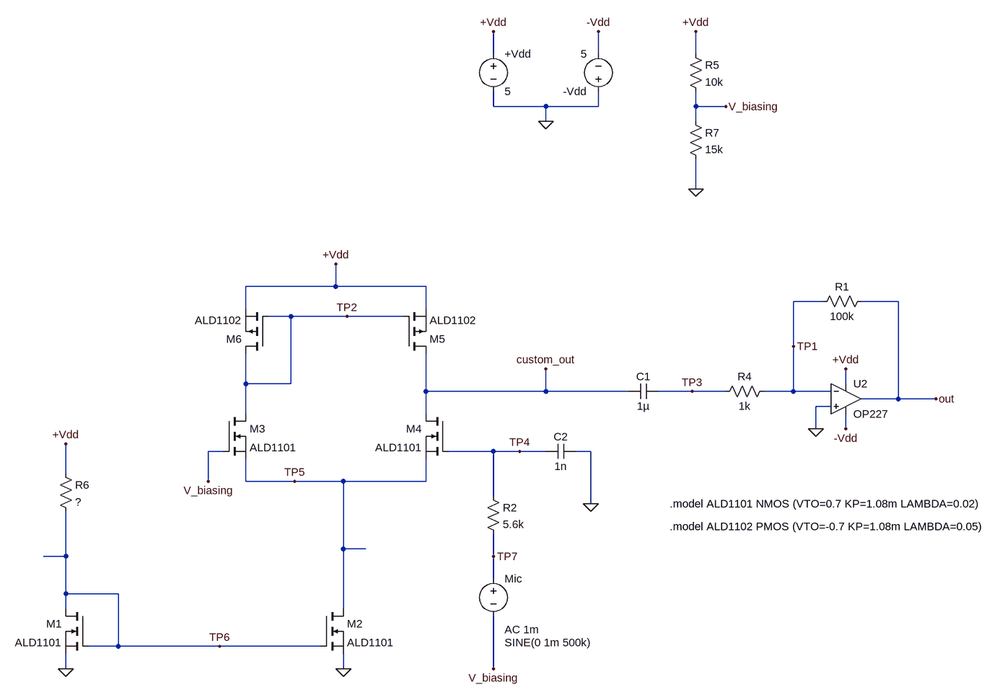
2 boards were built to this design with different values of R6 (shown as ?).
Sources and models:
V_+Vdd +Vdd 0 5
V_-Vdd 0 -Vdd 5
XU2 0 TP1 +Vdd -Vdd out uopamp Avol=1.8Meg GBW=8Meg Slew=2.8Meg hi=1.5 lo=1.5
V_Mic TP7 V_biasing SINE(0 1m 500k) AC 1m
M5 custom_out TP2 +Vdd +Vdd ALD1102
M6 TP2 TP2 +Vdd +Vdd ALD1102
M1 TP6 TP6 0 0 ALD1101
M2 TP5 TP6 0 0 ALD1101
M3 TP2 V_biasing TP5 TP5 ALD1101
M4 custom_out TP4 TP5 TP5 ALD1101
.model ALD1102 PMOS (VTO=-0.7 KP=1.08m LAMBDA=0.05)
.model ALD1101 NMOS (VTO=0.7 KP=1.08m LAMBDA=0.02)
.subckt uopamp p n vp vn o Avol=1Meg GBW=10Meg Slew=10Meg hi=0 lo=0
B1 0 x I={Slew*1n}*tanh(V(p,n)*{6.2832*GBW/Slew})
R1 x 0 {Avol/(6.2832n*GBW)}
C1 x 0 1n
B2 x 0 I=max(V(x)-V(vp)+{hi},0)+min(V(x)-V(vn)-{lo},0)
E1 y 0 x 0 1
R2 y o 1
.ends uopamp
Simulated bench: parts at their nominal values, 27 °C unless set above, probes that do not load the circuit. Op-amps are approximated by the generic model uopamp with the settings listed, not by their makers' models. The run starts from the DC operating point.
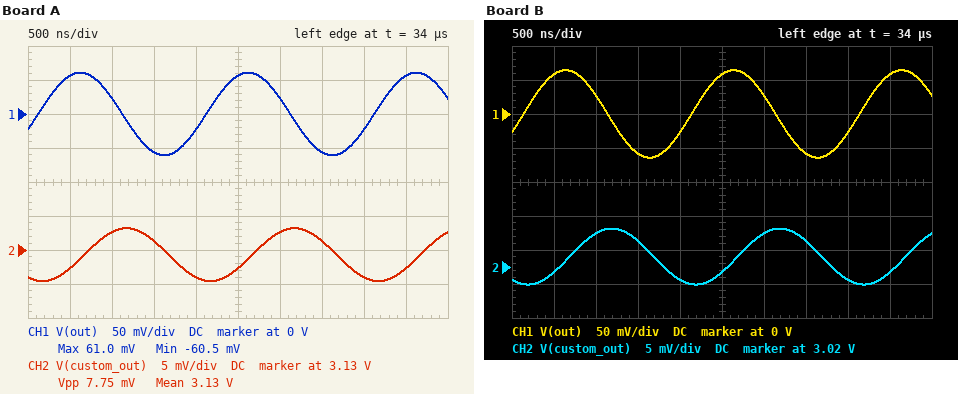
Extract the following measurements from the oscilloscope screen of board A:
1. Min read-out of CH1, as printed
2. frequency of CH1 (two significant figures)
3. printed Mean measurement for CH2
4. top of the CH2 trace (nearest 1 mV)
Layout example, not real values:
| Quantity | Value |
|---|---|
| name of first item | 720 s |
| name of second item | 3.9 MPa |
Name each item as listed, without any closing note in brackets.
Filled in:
| Quantity | Value |
|---|---|
| Min read-out of CH1, as printed | -60.5 mV |
| frequency of CH1 | 500 kHz |
| printed Mean measurement for CH2 | 3.13 V |
| top of the CH2 trace | 3.133 V |
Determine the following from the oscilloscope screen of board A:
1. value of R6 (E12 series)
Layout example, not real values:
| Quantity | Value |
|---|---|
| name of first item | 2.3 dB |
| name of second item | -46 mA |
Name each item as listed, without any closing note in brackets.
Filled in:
| Quantity | Value |
|---|---|
| value of R6 | 1.2 kΩ |
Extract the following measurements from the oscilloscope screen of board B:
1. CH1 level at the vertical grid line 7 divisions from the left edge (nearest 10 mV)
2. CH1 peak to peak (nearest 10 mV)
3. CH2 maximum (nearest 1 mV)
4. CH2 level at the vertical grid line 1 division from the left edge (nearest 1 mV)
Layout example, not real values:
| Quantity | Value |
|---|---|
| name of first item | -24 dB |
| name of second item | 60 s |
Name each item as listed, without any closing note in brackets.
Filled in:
| Quantity | Value |
|---|---|
| CH1 level at the vertical grid line 7 divisions from the left edge | -60 mV |
| CH1 peak to peak | 130 mV |
| CH2 maximum | 3.026 V |
| CH2 level at the vertical grid line 1 division from the left edge | 3.019 V |
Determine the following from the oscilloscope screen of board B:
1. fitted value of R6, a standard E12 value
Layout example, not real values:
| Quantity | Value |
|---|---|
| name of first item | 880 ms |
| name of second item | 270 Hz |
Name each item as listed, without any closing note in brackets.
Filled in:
| Quantity | Value |
|---|---|
| fitted value of R6, a standard E12 value | 680 Ω |
